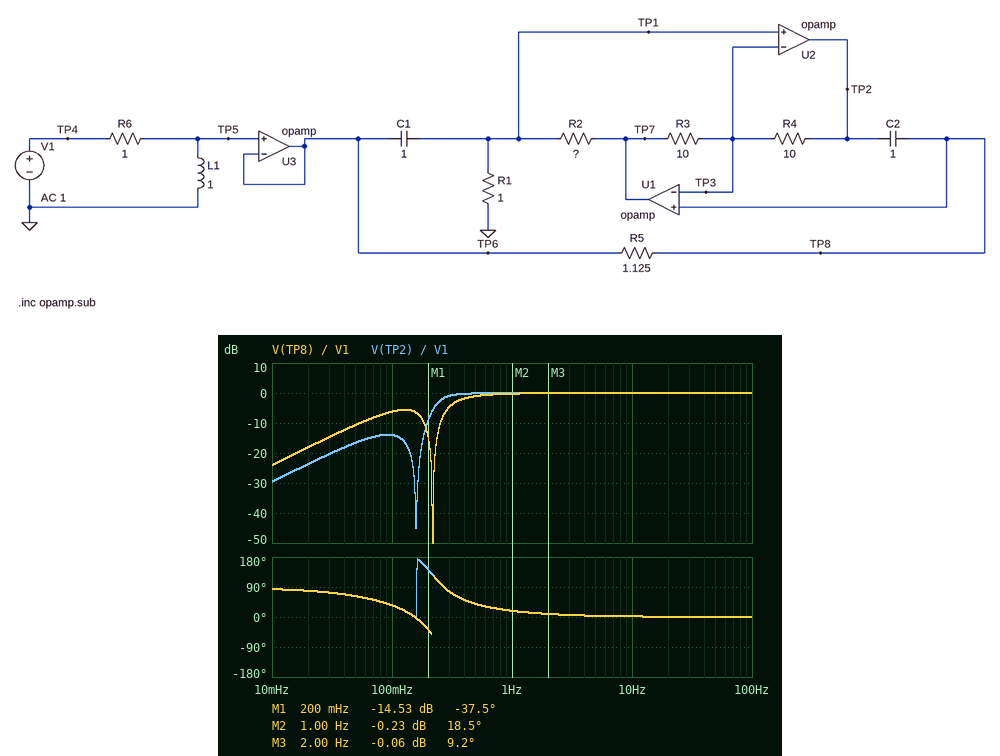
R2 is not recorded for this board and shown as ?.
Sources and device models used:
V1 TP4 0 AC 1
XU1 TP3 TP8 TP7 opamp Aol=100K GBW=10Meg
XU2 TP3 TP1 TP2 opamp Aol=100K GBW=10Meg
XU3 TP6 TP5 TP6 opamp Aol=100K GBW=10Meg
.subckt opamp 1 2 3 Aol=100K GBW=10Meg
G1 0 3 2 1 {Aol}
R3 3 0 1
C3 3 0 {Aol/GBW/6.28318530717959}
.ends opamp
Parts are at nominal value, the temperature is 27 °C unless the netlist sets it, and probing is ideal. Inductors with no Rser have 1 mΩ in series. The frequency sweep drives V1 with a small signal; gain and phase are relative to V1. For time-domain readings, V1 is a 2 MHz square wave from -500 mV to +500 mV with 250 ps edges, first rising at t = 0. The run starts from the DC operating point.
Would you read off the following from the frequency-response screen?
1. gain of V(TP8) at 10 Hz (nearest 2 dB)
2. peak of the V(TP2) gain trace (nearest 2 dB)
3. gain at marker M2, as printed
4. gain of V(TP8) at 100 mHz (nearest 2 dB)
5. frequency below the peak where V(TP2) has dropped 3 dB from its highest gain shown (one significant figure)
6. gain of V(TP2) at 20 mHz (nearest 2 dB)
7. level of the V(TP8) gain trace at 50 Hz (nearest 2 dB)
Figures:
0 dB
0 dB
-0.23 dB
-6 dB
200 mHz
-24 dB
0 dB
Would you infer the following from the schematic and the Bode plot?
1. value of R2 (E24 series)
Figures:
0.47 Ω
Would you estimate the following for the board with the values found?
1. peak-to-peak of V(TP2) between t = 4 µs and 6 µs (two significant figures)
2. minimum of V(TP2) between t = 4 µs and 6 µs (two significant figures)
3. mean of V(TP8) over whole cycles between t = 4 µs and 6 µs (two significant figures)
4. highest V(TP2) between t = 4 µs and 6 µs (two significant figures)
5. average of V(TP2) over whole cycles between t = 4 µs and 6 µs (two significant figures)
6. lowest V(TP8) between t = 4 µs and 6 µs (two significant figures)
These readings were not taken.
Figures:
1.3 V
-140 mV
500 mV
1.1 V
500 mV
-140 mV
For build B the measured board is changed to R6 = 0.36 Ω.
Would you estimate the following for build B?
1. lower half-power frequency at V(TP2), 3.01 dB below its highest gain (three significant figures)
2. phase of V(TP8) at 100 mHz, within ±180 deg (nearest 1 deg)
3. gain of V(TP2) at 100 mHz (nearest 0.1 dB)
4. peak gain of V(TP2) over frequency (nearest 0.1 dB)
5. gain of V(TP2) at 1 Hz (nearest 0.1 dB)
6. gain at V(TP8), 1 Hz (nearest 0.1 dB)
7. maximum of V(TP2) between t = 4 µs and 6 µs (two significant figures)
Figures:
231 mHz
7 deg
-9.8 dB
0.3 dB
0.1 dB
-0.1 dB
1.1 V
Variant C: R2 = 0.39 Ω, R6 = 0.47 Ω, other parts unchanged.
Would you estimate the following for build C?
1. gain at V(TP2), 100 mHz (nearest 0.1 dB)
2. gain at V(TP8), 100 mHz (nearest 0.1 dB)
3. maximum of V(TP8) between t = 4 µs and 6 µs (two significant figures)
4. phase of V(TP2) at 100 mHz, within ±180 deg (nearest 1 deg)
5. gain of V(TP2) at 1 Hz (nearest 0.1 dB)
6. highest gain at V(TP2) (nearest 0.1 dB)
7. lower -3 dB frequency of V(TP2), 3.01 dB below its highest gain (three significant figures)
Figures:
-7.9 dB
-2.4 dB
1.1 V
18 deg
0.1 dB
0.2 dB
259 mHz
